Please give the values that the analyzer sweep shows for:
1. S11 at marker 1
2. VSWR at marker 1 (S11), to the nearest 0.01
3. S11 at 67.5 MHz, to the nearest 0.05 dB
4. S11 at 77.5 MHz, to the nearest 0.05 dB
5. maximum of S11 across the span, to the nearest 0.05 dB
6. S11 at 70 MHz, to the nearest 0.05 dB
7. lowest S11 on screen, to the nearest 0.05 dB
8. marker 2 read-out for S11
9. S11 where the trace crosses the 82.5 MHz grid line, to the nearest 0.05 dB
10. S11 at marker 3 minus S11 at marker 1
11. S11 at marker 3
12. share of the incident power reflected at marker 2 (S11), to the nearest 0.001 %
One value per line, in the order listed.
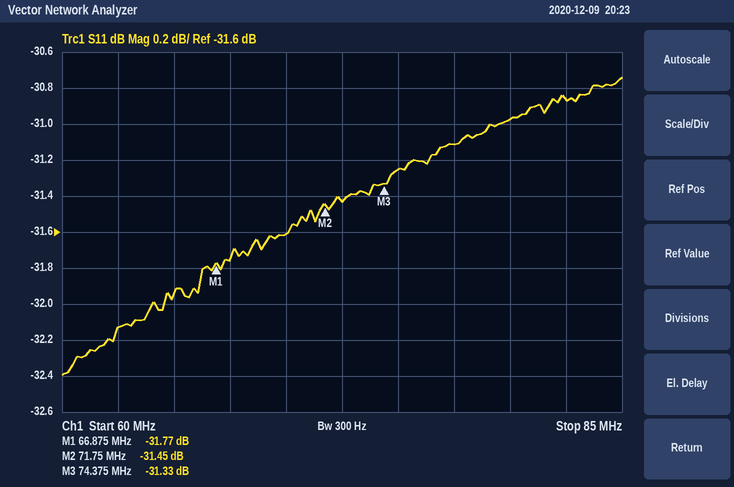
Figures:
-31.77 dB
1.05
-31.75 dB
-31.10 dB
-30.75 dB
-31.60 dB
-32.40 dB
-31.45 dB
-30.85 dB
0.44 dB
-31.33 dB
0.072 %
